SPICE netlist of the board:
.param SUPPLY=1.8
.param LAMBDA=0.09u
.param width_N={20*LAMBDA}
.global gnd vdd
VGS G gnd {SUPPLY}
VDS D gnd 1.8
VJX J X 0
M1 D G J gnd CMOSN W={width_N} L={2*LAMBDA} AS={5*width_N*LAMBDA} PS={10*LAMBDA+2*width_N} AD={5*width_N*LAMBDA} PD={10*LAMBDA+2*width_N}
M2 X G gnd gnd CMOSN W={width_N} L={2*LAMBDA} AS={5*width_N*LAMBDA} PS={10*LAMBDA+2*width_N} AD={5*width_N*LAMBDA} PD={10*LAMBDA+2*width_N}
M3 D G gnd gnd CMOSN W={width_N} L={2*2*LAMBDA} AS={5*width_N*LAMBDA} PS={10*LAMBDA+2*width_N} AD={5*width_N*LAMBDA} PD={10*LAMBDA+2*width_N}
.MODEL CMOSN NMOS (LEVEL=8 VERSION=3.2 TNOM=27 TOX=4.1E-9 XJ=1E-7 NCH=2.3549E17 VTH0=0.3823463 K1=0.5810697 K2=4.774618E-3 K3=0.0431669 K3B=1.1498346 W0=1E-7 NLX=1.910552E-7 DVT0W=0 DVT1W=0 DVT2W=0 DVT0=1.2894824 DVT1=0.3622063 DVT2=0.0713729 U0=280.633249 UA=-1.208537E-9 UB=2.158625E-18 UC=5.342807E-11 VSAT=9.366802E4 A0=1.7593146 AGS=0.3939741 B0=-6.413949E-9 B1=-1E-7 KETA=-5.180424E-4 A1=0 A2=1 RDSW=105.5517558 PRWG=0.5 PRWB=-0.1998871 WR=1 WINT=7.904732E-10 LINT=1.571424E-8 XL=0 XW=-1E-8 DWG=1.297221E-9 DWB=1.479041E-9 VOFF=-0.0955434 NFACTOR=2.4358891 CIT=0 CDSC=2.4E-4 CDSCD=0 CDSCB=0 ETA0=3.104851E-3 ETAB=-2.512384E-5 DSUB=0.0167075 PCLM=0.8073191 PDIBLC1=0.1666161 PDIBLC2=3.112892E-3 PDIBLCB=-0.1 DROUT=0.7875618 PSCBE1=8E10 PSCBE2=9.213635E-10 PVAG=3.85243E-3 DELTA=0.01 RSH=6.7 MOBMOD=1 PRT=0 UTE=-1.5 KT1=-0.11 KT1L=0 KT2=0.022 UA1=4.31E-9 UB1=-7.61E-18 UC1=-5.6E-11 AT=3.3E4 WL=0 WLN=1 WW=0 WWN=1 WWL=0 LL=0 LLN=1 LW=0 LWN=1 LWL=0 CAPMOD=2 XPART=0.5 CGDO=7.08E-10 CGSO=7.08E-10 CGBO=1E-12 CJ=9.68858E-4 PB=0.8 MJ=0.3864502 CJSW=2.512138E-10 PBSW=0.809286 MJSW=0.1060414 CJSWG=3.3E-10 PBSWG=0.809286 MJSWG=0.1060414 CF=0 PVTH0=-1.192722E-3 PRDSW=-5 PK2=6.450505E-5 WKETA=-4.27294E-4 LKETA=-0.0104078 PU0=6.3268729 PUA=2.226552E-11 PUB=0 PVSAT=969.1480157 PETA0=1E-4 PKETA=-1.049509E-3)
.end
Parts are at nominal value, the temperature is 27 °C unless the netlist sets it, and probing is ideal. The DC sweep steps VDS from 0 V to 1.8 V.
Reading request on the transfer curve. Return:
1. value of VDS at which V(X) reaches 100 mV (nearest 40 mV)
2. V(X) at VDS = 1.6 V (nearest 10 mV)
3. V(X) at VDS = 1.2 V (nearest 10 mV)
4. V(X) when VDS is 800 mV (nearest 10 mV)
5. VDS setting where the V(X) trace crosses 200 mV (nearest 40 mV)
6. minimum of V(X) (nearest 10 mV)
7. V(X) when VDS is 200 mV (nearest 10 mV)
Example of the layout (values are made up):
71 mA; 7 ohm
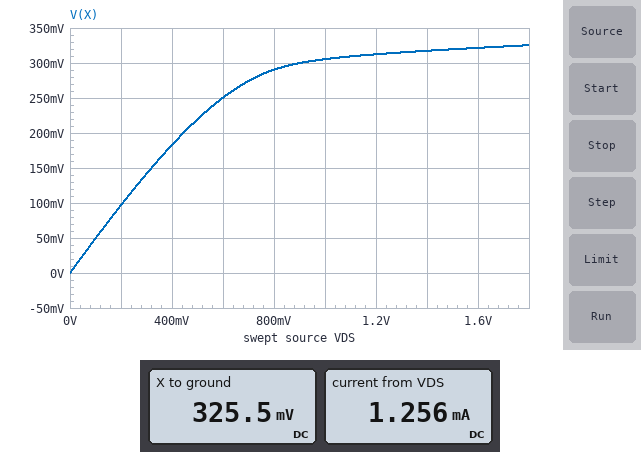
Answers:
200 mV; 320 mV; 310 mV; 290 mV; 440 mV; 0 V; 100 mV
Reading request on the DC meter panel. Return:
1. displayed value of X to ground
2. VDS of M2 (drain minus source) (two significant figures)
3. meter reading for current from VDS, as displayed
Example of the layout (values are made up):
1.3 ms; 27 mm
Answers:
325.5 mV; 330 mV; 1.256 mA
